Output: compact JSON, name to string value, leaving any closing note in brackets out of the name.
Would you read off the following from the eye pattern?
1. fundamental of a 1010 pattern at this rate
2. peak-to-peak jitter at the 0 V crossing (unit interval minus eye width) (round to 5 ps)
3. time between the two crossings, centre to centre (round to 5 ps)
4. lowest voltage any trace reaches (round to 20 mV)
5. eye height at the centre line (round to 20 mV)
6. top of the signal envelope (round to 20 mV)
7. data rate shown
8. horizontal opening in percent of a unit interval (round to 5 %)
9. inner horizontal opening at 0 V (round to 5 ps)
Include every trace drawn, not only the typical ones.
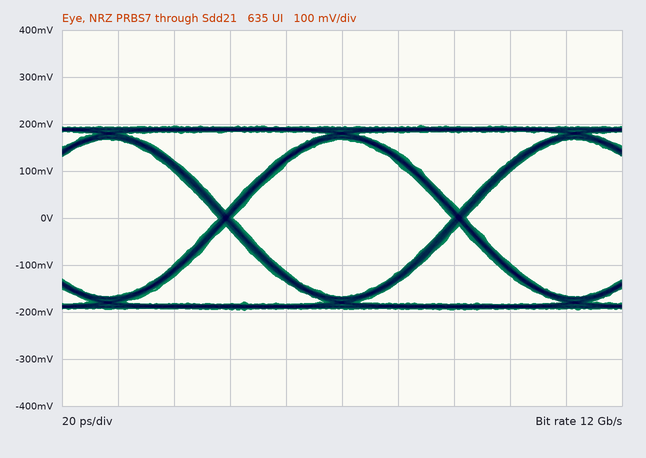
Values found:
{"fundamental of a 1010 pattern at this rate": "6 GHz", "peak-to-peak jitter at the 0 V crossing (unit interval minus eye width)": "5 ps", "time between the two crossings, centre to centre": "85 ps", "lowest voltage any trace reaches": "-200 mV", "eye height at the centre line": "340 mV", "top of the signal envelope": "200 mV", "data rate shown": "12 Gb/s", "horizontal opening in percent of a unit interval": "95 %", "inner horizontal opening at 0 V": "80 ps"}
